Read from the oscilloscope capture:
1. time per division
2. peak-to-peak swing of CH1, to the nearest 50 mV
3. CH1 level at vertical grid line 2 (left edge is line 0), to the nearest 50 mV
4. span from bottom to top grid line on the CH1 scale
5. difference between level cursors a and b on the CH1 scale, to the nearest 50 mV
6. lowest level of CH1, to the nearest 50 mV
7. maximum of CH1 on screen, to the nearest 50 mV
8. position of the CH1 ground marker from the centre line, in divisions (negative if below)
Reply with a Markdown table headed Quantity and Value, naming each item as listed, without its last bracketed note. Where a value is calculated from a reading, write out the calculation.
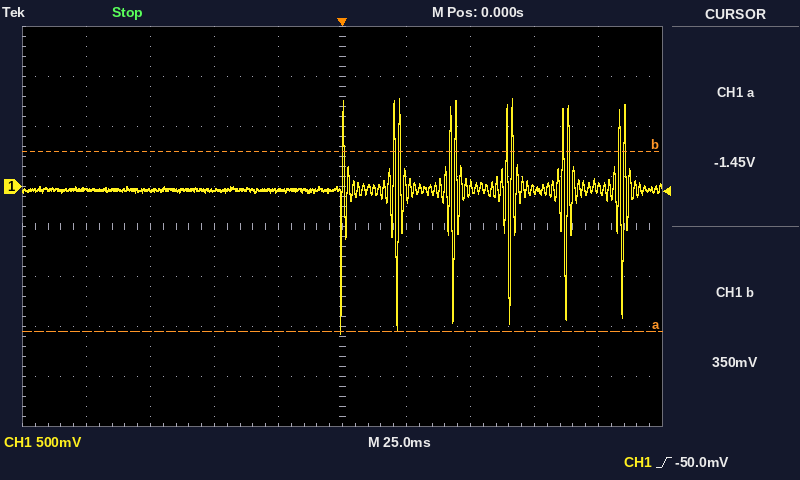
| Quantity | Value |
|---|---|
| time per division | 25 ms |
| peak-to-peak swing of CH1, to the nearest 50 mV | 900 mV − (-1.45 V) = 2.35 V |
| CH1 level at vertical grid line 2 (left edge is line 0), to the nearest 50 mV | -50 mV |
| span from bottom to top grid line on the CH1 scale | 4 V |
| difference between level cursors a and b on the CH1 scale, to the nearest 50 mV | 1.80 V |
| lowest level of CH1, to the nearest 50 mV | -1.45 V |
| maximum of CH1 on screen, to the nearest 50 mV | 900 mV |
| position of the CH1 ground marker from the centre line, in divisions | +0.8 div |
